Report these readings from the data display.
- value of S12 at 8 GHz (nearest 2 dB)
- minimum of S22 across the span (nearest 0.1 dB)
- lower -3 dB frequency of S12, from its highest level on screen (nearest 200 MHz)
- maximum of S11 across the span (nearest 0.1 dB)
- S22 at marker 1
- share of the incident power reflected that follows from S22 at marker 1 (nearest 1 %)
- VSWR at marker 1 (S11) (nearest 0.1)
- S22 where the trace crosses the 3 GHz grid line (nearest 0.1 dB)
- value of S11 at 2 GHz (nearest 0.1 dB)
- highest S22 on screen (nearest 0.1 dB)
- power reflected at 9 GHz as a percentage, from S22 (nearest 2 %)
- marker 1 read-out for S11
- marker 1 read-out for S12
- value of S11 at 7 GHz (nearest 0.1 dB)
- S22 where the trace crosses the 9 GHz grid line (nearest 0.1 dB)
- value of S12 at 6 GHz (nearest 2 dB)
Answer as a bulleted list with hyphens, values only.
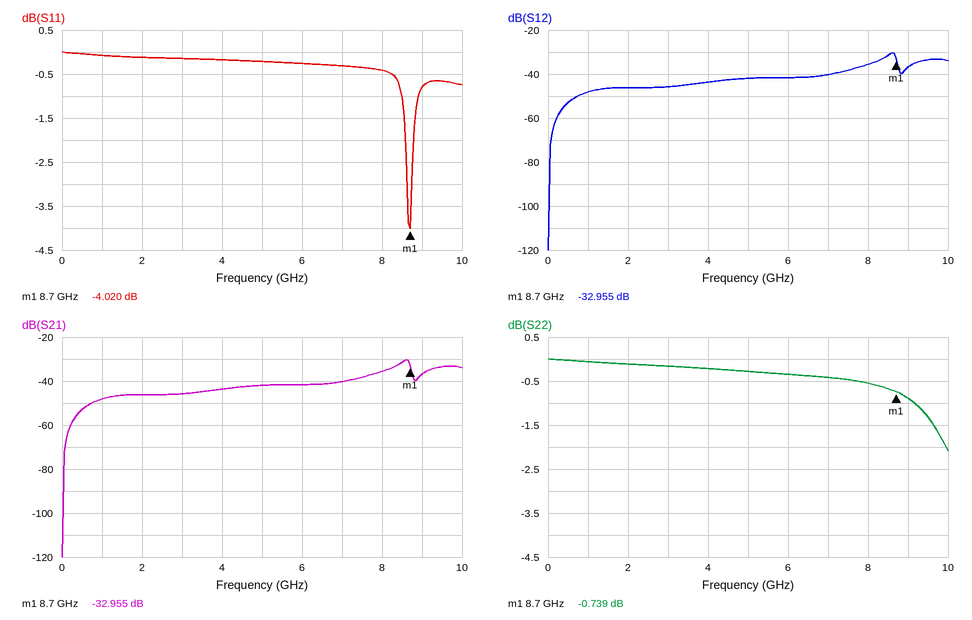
- -36 dB
- -2.1 dB
- 8.4 GHz
- 0.0 dB
- -0.739 dB
- 84 %
- 4.4
- -0.2 dB
- -0.1 dB
- 0.0 dB
- 82 %
- -4.020 dB
- -32.955 dB
- -0.3 dB
- -0.9 dB
- -42 dB
